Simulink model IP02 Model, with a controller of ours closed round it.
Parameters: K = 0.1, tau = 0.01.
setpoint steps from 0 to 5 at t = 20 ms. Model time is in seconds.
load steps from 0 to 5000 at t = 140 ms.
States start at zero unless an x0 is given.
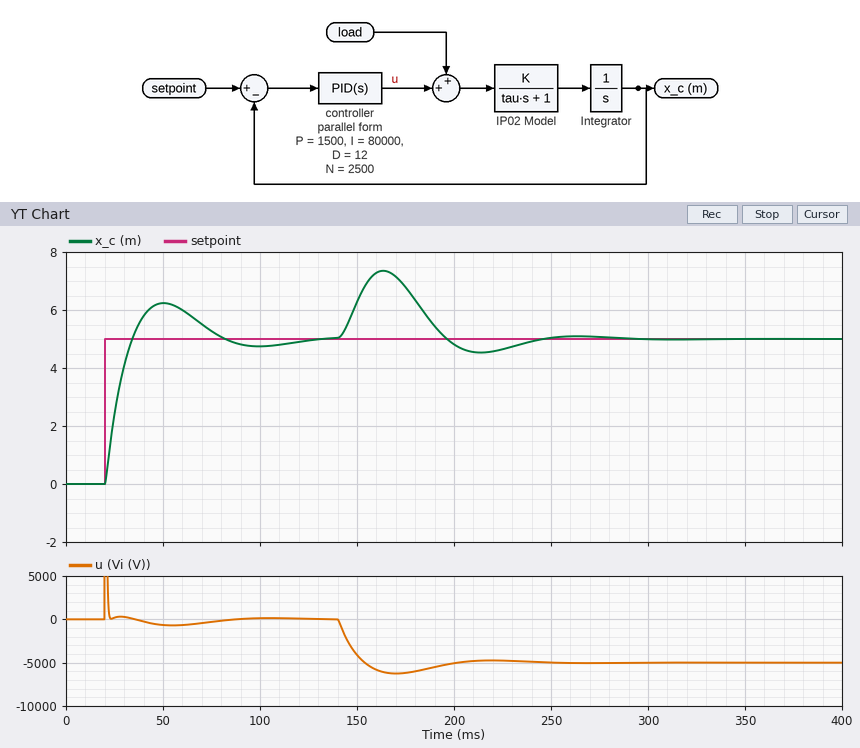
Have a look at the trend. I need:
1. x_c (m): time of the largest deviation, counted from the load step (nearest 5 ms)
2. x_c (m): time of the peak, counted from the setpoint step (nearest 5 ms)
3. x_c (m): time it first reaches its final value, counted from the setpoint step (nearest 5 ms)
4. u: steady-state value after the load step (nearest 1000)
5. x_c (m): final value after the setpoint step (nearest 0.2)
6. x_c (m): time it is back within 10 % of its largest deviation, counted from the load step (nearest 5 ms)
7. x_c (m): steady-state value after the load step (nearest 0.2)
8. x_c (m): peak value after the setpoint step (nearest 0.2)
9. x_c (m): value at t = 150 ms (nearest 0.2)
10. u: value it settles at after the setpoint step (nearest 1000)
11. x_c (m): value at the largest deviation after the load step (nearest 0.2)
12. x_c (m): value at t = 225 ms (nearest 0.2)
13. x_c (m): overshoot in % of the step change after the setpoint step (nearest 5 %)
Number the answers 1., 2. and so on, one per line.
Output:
1. 25 ms
2. 30 ms
3. 15 ms
4. -5000
5. 5.0
6. 90 ms
7. 5.0
8. 6.2
9. 6.2
10. 0
11. 7.4
12. 4.6
13. 25 %
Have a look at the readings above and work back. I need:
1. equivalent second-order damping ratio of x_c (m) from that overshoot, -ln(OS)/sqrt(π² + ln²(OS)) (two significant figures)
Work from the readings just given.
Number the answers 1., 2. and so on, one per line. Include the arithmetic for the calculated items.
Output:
1. ln(0.25) = -1.386; 1.386 / sqrt(9.870 + 1.922) = 0.40
